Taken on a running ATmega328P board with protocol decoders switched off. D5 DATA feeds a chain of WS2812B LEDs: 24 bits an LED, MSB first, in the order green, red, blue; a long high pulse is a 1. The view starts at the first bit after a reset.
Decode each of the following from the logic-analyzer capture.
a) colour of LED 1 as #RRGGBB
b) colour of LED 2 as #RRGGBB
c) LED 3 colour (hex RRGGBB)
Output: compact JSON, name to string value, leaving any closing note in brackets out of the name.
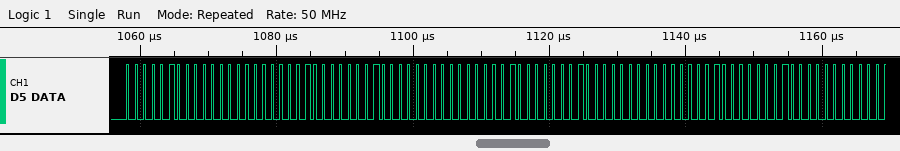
{"colour of LED 1 as #RRGGBB": "#000404", "colour of LED 2 as #RRGGBB": "#000404", "LED 3 colour": "#000404"}
